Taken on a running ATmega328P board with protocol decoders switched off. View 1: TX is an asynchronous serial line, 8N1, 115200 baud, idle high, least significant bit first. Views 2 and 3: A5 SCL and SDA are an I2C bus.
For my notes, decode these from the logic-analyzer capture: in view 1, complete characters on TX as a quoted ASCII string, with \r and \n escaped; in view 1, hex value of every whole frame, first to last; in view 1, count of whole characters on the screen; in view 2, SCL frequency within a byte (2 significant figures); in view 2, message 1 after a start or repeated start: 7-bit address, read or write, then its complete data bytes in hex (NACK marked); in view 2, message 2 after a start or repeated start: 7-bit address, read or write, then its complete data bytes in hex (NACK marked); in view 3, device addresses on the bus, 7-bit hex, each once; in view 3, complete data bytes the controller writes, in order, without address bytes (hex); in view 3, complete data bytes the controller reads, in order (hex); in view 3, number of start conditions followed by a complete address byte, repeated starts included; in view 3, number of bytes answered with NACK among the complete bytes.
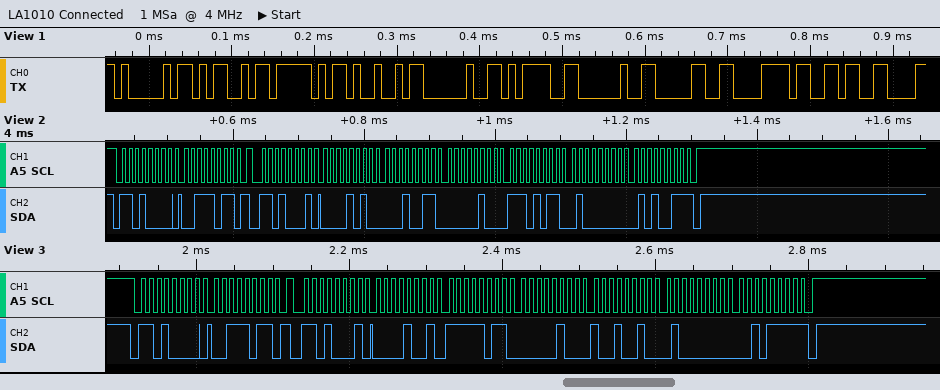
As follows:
"AM_I = 0x6"
0x41 0x4D 0x5F 0x49 0x20 0x3D 0x20 0x30 0x78 0x36
10
100 kHz
0x68 write: 3B
0x68 read: 0A 13 04 EB 40 53 NACK
0x68
3B
09 FB 04 92 40 2F
2
1
